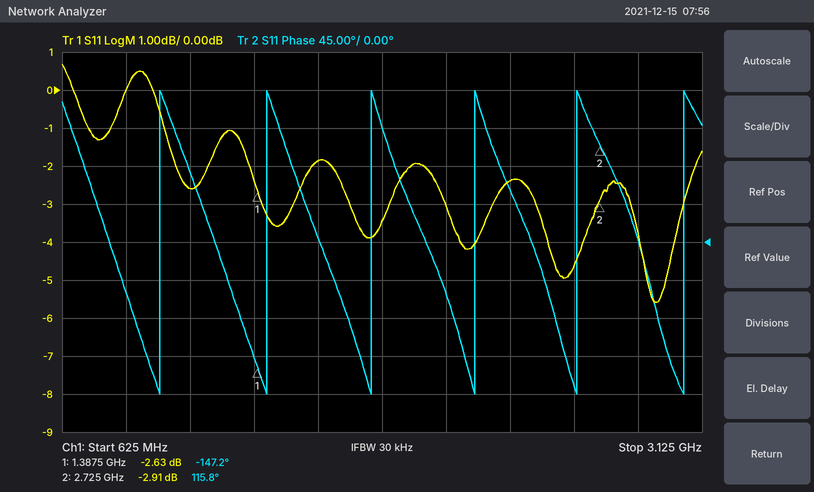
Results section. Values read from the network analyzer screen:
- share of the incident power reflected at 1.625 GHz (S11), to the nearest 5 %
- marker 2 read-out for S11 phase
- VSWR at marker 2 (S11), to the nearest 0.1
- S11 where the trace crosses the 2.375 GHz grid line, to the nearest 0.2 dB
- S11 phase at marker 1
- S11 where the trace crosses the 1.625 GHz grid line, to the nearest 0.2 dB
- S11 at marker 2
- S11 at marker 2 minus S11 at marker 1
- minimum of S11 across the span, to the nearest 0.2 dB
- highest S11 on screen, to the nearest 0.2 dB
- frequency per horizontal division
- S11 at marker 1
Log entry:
65 %
115.8°
6.0
-2.4 dB
-147.2°
-1.8 dB
-2.91 dB
-0.28 dB
-5.6 dB
0.6 dB
250 MHz
-2.63 dB
